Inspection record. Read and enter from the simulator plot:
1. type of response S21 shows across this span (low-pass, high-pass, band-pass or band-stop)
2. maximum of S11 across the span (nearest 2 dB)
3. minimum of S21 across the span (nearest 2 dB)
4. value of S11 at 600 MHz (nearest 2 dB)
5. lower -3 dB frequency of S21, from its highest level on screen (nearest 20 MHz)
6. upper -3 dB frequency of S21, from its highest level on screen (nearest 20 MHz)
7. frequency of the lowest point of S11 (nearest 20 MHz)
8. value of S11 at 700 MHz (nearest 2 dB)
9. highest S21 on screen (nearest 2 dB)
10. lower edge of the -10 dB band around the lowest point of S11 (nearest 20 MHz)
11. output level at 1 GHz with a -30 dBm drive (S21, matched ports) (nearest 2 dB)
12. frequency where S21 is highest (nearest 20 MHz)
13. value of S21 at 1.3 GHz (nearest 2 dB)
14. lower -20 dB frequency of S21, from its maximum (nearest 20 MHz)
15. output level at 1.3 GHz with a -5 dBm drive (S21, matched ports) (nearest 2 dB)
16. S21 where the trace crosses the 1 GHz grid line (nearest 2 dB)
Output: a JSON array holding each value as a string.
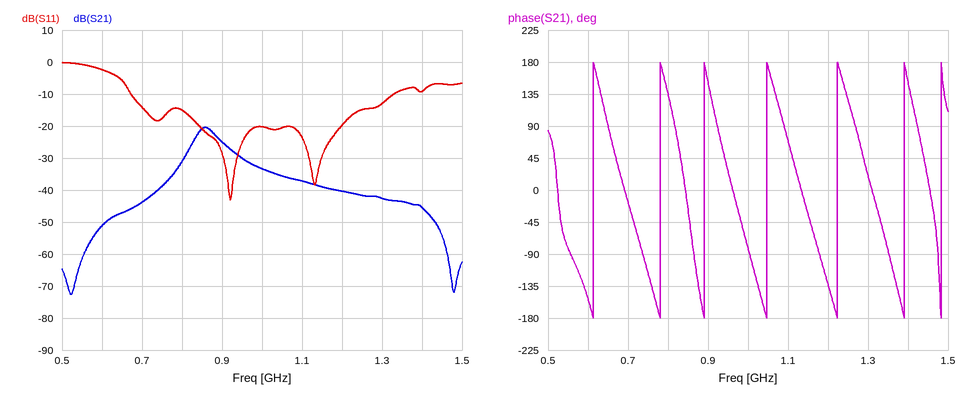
["band-pass", "0 dB", "-72 dB", "-2 dB", "840 MHz", "880 MHz", "920 MHz", "-14 dB", "-20 dB", "680 MHz", "-64 dBm", "860 MHz", "-42 dB", "740 MHz", "-48 dBm", "-34 dB"]
